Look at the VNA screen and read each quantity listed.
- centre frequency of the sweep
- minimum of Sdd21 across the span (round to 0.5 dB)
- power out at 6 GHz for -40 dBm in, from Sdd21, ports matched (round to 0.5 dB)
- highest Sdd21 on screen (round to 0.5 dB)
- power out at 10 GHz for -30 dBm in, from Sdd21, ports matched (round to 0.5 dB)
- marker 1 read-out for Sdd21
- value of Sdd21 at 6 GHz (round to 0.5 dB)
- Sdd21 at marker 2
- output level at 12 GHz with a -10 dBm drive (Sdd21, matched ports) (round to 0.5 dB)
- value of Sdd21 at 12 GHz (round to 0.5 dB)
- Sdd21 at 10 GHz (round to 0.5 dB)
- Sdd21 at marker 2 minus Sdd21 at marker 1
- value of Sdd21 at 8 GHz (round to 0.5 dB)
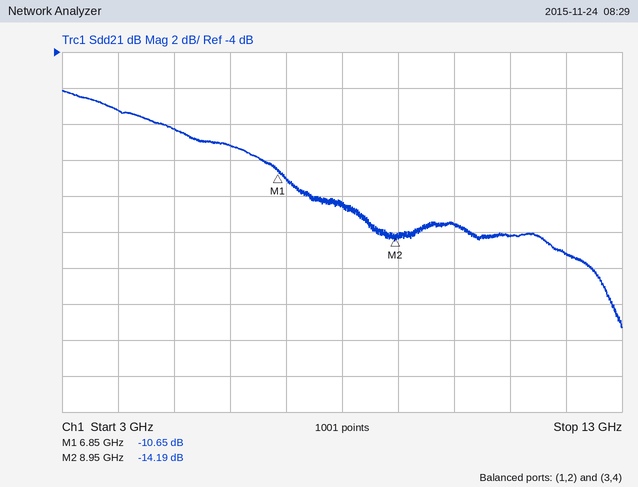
8 GHz
-19.5 dB
-49.0 dBm
-6.0 dB
-43.5 dBm
-10.65 dB
-9.0 dB
-14.19 dB
-25.0 dBm
-15.0 dB
-13.5 dB
-3.54 dB
-12.5 dB
